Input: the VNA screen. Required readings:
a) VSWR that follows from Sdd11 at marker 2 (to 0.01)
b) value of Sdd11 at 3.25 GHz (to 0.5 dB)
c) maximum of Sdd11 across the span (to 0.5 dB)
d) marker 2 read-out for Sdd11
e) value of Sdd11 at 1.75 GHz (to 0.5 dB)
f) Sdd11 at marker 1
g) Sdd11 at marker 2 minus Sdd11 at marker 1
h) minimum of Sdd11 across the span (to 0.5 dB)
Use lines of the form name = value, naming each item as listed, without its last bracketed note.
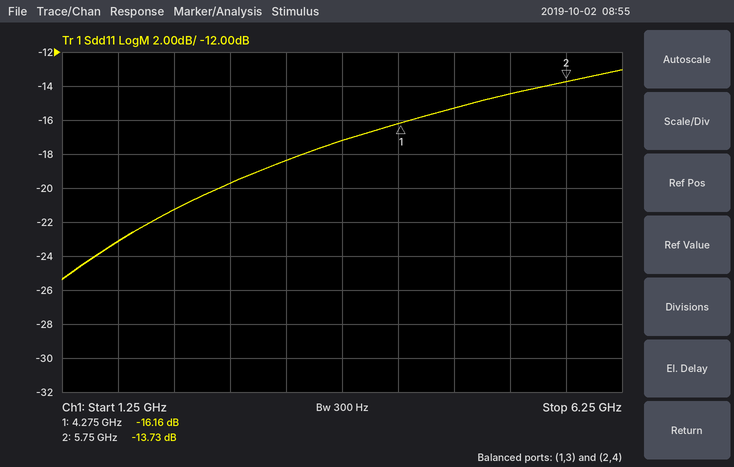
VSWR that follows from Sdd11 at marker 2 = 1.52
value of Sdd11 at 3.25 GHz = -18.5 dB
maximum of Sdd11 across the span = -13.0 dB
marker 2 read-out for Sdd11 = -13.73 dB
value of Sdd11 at 1.75 GHz = -23.0 dB
Sdd11 at marker 1 = -16.16 dB
Sdd11 at marker 2 minus Sdd11 at marker 1 = 2.43 dB
minimum of Sdd11 across the span = -25.5 dB
